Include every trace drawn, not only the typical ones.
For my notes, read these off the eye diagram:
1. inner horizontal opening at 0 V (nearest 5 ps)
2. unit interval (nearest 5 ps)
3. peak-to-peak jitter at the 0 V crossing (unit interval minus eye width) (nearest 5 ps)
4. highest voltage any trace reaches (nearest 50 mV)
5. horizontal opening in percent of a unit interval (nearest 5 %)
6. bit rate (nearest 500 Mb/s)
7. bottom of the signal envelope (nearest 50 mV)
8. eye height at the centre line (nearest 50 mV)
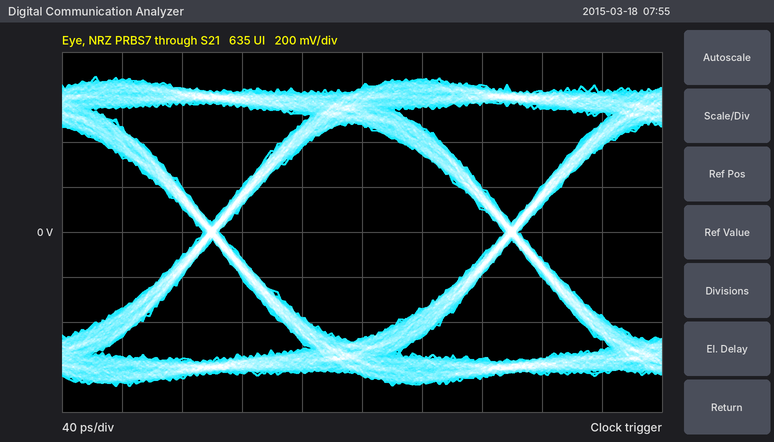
190 ps
200 ps
10 ps
700 mV
95 %
5.0 Gb/s
-700 mV
950 mV
